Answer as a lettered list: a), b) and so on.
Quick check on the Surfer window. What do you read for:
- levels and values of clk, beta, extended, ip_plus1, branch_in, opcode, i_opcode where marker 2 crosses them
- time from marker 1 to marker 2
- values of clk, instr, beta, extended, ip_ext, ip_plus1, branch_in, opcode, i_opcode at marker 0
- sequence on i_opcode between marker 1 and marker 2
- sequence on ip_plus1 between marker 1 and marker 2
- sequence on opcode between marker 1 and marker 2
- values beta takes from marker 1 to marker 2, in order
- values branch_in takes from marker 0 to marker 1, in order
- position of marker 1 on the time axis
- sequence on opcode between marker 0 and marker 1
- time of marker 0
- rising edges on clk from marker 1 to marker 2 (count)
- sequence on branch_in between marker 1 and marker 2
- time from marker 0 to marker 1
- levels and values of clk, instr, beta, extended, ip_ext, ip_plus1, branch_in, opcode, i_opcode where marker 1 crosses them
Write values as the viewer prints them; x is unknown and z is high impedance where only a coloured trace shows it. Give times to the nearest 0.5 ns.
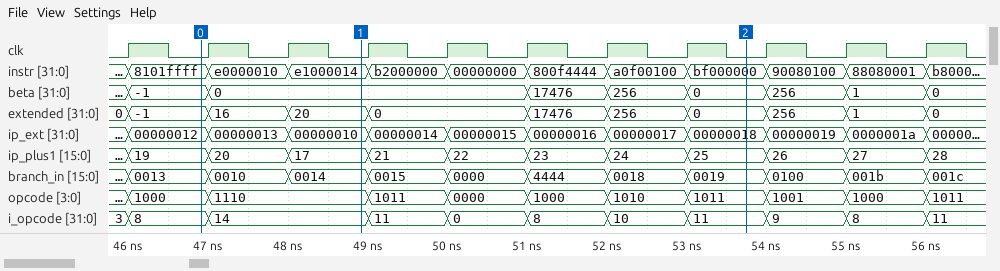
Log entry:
a) clk=0, beta=0, extended=0, ip_plus1=25, branch_in=0019, opcode=1011, i_opcode=11
b) 5 ns
c) clk=0, instr=8101ffff, beta=-1, extended=-1, ip_ext=00000012, ip_plus1=19, branch_in=0013, opcode=1000, i_opcode=8
d) 14, 11, 0, 8, 10, 11
e) 17, 21, 22, 23, 24, 25
f) 1110, 1011, 0000, 1000, 1010, 1011
g) 0, 17476, 256, 0
h) 0013, 0010, 0014
i) 49 ns
j) 1000, 1110
k) 47 ns
l) 5
m) 0014, 0015, 0000, 4444, 0018, 0019
n) 2 ns
o) clk=0, instr=e1000014, beta=0, extended=20, ip_ext=00000010, ip_plus1=17, branch_in=0014, opcode=1110, i_opcode=14
